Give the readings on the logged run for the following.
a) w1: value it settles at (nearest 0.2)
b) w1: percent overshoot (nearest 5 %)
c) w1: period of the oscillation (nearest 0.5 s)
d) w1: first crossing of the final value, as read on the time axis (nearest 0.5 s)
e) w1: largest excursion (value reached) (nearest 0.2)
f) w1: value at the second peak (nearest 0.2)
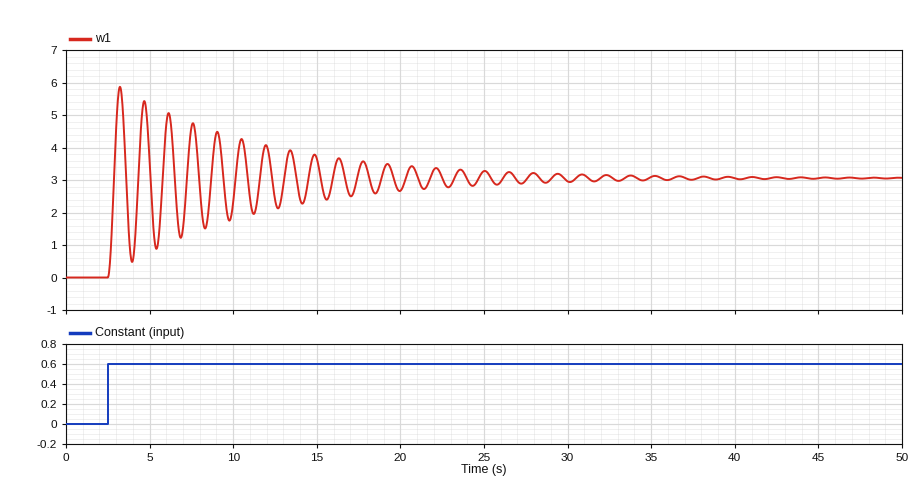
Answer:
3.0
90 %
1.5 s
3.0 s
5.8
5.4
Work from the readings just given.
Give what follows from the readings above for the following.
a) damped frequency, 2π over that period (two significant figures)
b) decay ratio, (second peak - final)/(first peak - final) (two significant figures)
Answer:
4.2 rad/s
0.86
